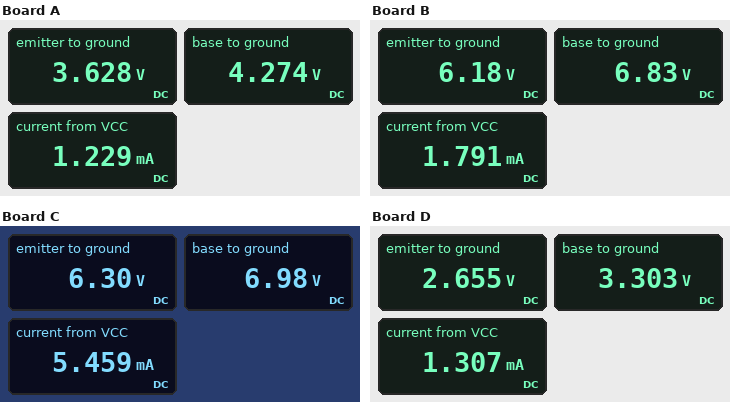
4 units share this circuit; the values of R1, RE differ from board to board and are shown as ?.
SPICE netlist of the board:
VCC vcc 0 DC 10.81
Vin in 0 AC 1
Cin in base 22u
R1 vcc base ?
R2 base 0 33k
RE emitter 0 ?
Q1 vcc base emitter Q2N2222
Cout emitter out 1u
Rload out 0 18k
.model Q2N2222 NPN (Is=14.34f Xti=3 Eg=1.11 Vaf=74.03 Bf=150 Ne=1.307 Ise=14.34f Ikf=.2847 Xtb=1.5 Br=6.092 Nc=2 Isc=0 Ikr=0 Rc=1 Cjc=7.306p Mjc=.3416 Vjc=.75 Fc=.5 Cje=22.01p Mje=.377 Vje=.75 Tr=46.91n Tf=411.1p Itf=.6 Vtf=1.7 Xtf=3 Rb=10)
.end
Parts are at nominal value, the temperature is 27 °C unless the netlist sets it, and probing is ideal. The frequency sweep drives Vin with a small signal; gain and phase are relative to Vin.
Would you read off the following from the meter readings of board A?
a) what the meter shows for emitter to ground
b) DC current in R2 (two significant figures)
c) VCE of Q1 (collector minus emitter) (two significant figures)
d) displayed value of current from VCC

3.628 V
130 µA
7.2 V
1.229 mA
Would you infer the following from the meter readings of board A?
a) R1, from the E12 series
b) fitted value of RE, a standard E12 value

47 kΩ
3.3 kΩ
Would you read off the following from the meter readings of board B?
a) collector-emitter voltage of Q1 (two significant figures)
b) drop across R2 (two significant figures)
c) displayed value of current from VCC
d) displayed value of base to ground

4.6 V
6.8 V
1.791 mA
6.83 V
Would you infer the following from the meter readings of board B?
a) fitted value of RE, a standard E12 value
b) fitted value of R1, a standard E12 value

3.9 kΩ
18 kΩ
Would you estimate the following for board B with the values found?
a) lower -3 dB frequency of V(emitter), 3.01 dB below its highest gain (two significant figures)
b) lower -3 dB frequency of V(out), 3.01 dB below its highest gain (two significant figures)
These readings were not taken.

640 mHz
8.9 Hz
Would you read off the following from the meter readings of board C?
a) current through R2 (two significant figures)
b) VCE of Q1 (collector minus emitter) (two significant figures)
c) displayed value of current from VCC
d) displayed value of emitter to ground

210 µA
4.5 V
5.459 mA
6.30 V
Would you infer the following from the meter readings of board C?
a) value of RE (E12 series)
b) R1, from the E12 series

1.2 kΩ
15 kΩ
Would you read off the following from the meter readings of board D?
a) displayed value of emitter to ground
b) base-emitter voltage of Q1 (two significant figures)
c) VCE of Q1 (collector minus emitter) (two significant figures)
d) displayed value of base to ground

2.655 V
650 mV
8.2 V
3.303 V
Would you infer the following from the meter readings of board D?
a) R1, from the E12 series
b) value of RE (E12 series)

68 kΩ
2.2 kΩ
